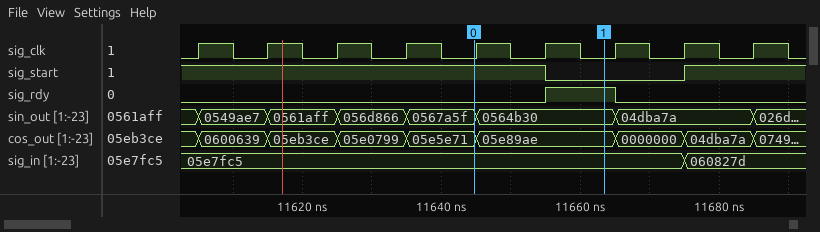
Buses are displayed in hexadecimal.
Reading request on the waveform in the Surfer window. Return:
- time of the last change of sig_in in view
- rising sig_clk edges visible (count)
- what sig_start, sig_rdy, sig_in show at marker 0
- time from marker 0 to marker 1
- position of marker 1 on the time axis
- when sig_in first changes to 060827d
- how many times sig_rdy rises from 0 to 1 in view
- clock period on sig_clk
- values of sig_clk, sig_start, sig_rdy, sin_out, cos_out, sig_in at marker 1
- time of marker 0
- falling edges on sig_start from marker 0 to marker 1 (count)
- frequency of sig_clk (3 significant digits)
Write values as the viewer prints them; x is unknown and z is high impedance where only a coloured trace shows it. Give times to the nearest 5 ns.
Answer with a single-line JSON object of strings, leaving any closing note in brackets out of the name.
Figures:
{"time of the last change of sig_in in view": "11675 ns", "rising sig_clk edges visible": "9", "what sig_start, sig_rdy, sig_in show at marker 0": "sig_start=1, sig_rdy=0, sig_in=05e7fc5", "time from marker 0 to marker 1": "20 ns", "position of marker 1 on the time axis": "11665 ns", "when sig_in first changes to 060827d": "11675 ns", "how many times sig_rdy rises from 0 to 1 in view": "1", "clock period on sig_clk": "10 ns", "values of sig_clk, sig_start, sig_rdy, sin_out, cos_out, sig_in at marker 1": "sig_clk=0, sig_start=0, sig_rdy=1, sin_out=0564b30, cos_out=05e89ae, sig_in=05e7fc5", "time of marker 0": "11645 ns", "falling edges on sig_start from marker 0 to marker 1": "1", "frequency of sig_clk": "100 MHz"}
